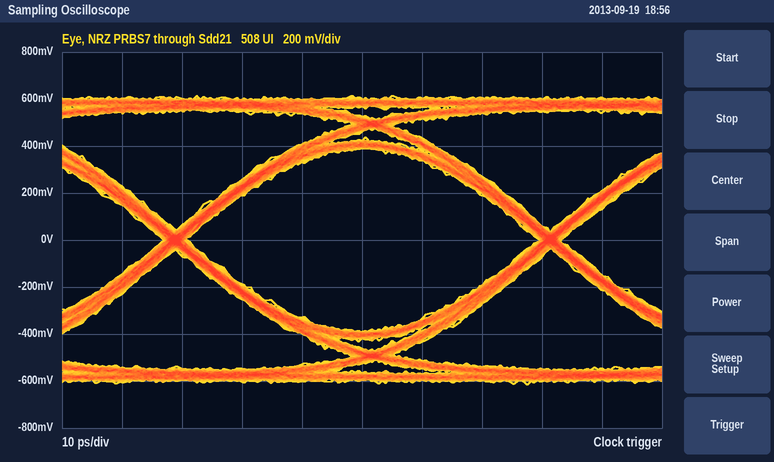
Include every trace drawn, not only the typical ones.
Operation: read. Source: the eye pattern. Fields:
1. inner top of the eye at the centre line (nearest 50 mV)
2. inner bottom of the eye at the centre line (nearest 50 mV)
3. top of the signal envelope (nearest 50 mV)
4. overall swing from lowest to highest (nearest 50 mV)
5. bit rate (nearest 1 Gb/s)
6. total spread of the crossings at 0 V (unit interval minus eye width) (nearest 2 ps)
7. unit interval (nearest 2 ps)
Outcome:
400 mV
-400 mV
600 mV
1.25 V
16 Gb/s
4 ps
62 ps
